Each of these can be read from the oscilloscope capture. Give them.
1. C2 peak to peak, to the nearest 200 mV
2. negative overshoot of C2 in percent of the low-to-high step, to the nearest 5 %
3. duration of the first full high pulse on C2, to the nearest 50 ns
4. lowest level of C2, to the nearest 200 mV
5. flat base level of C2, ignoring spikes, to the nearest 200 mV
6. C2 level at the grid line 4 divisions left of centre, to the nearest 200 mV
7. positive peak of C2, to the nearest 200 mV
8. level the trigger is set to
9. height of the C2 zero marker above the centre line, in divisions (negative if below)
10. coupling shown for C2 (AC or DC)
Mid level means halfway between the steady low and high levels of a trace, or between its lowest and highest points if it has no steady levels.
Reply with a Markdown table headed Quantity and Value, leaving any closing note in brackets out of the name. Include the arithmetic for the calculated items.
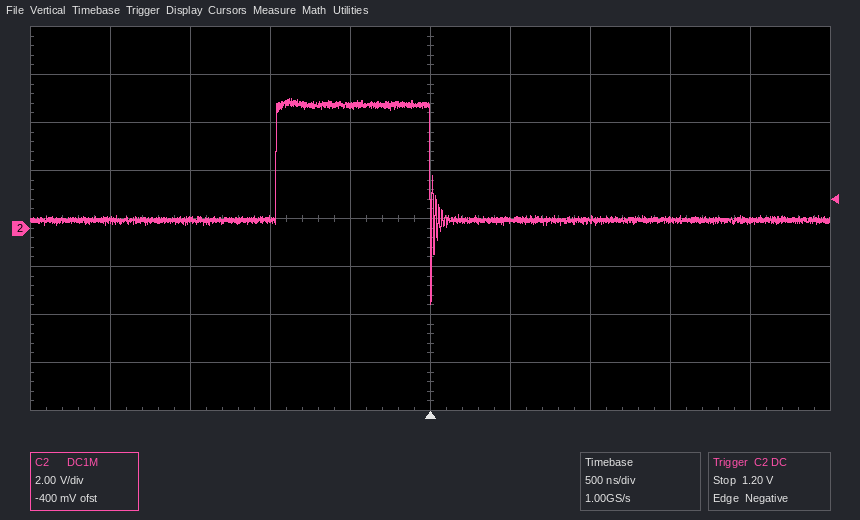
| Quantity | Value |
|---|---|
| C2 peak to peak, to the nearest 200 mV | 5.4 V − (-3.2 V) = 8.6 V |
| negative overshoot of C2 in percent of the low-to-high step, to the nearest 5 % | 75 % |
| duration of the first full high pulse on C2, to the nearest 50 ns | 950 ns |
| lowest level of C2, to the nearest 200 mV | -3.2 V |
| flat base level of C2, ignoring spikes, to the nearest 200 mV | 400 mV |
| C2 level at the grid line 4 divisions left of centre, to the nearest 200 mV | 400 mV |
| positive peak of C2, to the nearest 200 mV | 5.4 V |
| level the trigger is set to | 1.20 V |
| height of the C2 zero marker above the centre line, in divisions | -0.2 div |
| coupling shown for C2 | DC |
